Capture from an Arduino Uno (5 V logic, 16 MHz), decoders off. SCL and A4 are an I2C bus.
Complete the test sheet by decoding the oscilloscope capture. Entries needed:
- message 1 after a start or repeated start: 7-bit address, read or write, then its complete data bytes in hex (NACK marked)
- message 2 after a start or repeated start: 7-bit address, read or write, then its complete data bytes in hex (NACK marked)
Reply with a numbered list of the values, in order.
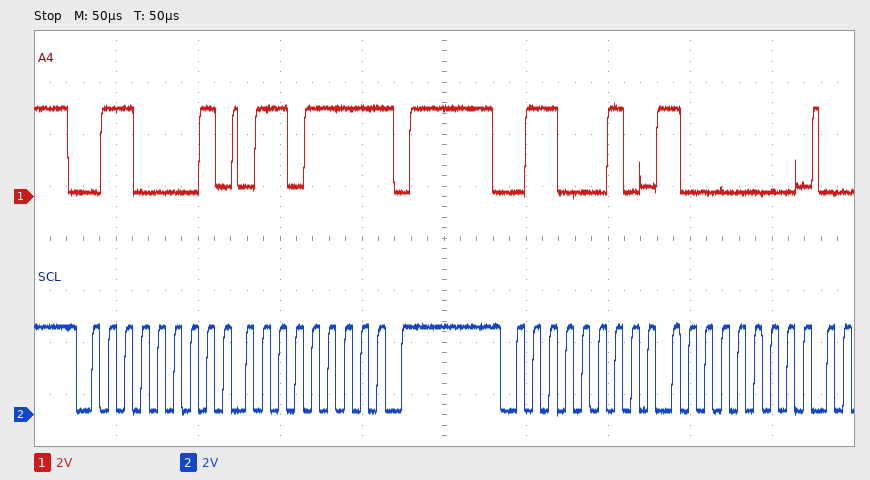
1. 0x30 read: 6F NACK
2. 0x31 write: 80
